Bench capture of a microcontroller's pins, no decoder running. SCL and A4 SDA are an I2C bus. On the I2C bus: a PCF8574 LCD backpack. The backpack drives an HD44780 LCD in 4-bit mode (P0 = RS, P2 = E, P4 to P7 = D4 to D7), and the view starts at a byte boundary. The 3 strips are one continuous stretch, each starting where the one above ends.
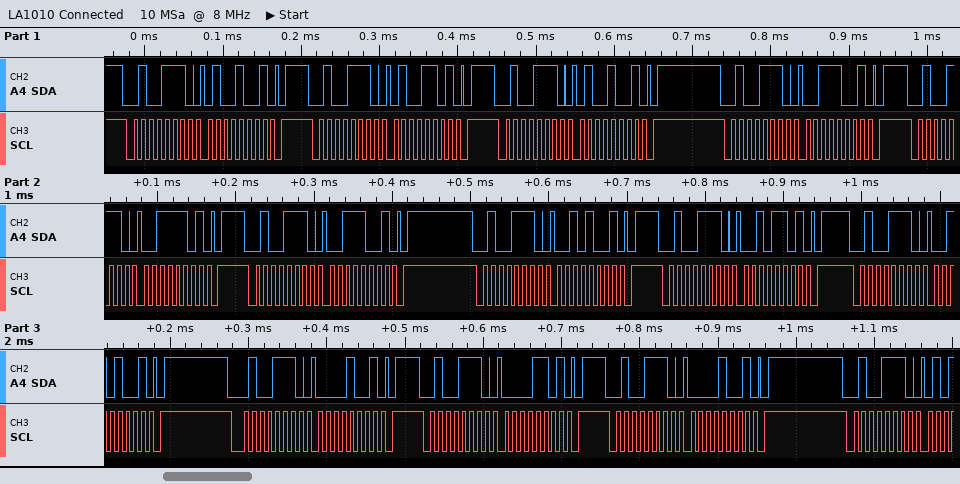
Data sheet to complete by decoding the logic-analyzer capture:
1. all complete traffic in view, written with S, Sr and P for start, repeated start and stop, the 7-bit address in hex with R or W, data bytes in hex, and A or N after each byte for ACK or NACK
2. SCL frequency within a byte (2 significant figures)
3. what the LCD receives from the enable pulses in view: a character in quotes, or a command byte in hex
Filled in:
S 27W A 49 A P S 27W A 4D A P S 27W A 49 A P S 27W A 39 A P S 27W A 3D A P S 27W A 39 A P S 27W A 29 A P S 27W A 2D A P S 27W A 29 A P S 27W A 09 A P S 27W A 0D A P S 27W A 09 A P S 27W A
100 kHz
'C' ' '
